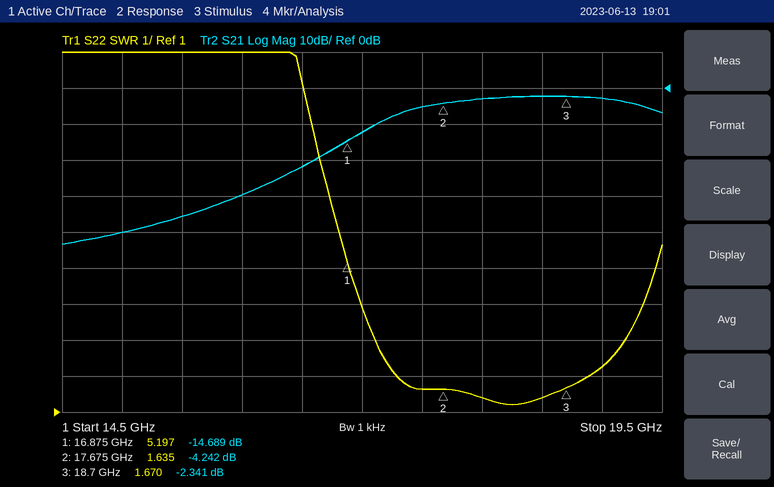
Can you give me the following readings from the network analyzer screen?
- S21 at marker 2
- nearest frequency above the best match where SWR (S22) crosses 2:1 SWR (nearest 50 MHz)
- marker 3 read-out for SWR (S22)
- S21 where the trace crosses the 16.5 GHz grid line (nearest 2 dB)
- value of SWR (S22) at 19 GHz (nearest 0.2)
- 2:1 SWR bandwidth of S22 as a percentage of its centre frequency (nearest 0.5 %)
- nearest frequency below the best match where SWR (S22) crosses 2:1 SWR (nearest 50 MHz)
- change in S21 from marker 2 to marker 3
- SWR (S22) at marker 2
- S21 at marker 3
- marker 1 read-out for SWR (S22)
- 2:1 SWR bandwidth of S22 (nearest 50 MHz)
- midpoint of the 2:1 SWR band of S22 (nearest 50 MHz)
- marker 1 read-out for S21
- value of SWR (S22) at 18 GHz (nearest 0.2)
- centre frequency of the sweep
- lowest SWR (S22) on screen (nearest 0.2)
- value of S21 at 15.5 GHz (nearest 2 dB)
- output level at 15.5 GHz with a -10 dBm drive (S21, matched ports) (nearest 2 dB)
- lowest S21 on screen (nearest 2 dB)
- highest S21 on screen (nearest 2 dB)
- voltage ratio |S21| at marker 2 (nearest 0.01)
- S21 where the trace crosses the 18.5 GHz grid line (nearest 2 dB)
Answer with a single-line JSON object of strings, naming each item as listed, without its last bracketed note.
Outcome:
{"S21 at marker 2": "-4.242 dB", "nearest frequency above the best match where SWR (S22) crosses 2:1 SWR": "18.90 GHz", "marker 3 read-out for SWR": "1.670", "S21 where the trace crosses the 16.5 GHz grid line": "-22 dB", "value of SWR (S22) at 19 GHz": "2.2", "2:1 SWR bandwidth of S22 as a percentage of its centre frequency": "9.0 %", "nearest frequency below the best match where SWR (S22) crosses 2:1 SWR": "17.30 GHz", "change in S21 from marker 2 to marker 3": "1.901 dB", "SWR (S22) at marker 2": "1.635", "S21 at marker 3": "-2.341 dB", "marker 1 read-out for SWR": "5.197", "2:1 SWR bandwidth of S22": "1.60 GHz", "midpoint of the 2:1 SWR band of S22": "18.10 GHz", "marker 1 read-out for S21": "-14.689 dB", "value of SWR (S22) at 18 GHz": "1.4", "centre frequency of the sweep": "17 GHz", "lowest SWR (S22) on screen": "1.2", "value of S21 at 15.5 GHz": "-36 dB", "output level at 15.5 GHz with a -10 dBm drive (S21, matched ports)": "-46 dBm", "lowest S21 on screen": "-44 dB", "highest S21 on screen": "-2 dB", "voltage ratio |S21| at marker 2": "0.61", "S21 where the trace crosses the 18.5 GHz grid line": "-2 dB"}
